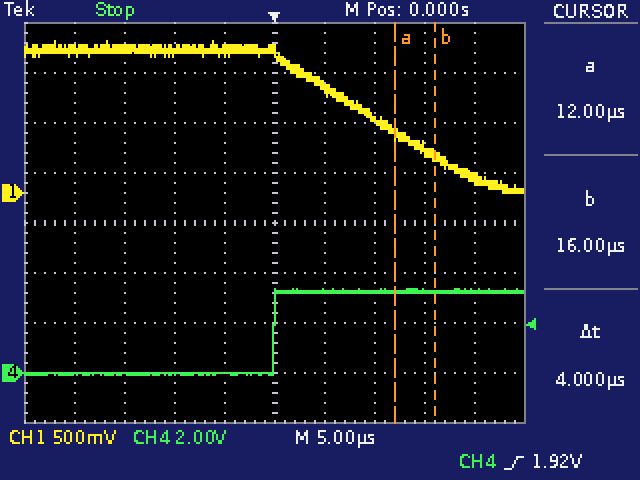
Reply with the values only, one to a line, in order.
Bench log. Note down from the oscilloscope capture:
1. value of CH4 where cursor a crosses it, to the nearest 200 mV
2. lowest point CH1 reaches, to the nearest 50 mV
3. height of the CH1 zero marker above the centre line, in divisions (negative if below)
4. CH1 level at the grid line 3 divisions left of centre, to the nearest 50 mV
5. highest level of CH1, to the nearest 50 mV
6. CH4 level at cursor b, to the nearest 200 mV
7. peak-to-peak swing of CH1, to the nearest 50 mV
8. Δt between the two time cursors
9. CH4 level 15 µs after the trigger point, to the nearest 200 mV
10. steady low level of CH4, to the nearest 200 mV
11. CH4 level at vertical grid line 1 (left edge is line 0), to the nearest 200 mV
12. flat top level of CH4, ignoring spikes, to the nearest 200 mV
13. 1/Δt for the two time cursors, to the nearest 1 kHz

3.2 V
0 mV
+0.6 div
1.45 V
1.50 V
3.2 V
1.50 V
4 µs
3.2 V
0.0 V
0.0 V
3.2 V
250 kHz
